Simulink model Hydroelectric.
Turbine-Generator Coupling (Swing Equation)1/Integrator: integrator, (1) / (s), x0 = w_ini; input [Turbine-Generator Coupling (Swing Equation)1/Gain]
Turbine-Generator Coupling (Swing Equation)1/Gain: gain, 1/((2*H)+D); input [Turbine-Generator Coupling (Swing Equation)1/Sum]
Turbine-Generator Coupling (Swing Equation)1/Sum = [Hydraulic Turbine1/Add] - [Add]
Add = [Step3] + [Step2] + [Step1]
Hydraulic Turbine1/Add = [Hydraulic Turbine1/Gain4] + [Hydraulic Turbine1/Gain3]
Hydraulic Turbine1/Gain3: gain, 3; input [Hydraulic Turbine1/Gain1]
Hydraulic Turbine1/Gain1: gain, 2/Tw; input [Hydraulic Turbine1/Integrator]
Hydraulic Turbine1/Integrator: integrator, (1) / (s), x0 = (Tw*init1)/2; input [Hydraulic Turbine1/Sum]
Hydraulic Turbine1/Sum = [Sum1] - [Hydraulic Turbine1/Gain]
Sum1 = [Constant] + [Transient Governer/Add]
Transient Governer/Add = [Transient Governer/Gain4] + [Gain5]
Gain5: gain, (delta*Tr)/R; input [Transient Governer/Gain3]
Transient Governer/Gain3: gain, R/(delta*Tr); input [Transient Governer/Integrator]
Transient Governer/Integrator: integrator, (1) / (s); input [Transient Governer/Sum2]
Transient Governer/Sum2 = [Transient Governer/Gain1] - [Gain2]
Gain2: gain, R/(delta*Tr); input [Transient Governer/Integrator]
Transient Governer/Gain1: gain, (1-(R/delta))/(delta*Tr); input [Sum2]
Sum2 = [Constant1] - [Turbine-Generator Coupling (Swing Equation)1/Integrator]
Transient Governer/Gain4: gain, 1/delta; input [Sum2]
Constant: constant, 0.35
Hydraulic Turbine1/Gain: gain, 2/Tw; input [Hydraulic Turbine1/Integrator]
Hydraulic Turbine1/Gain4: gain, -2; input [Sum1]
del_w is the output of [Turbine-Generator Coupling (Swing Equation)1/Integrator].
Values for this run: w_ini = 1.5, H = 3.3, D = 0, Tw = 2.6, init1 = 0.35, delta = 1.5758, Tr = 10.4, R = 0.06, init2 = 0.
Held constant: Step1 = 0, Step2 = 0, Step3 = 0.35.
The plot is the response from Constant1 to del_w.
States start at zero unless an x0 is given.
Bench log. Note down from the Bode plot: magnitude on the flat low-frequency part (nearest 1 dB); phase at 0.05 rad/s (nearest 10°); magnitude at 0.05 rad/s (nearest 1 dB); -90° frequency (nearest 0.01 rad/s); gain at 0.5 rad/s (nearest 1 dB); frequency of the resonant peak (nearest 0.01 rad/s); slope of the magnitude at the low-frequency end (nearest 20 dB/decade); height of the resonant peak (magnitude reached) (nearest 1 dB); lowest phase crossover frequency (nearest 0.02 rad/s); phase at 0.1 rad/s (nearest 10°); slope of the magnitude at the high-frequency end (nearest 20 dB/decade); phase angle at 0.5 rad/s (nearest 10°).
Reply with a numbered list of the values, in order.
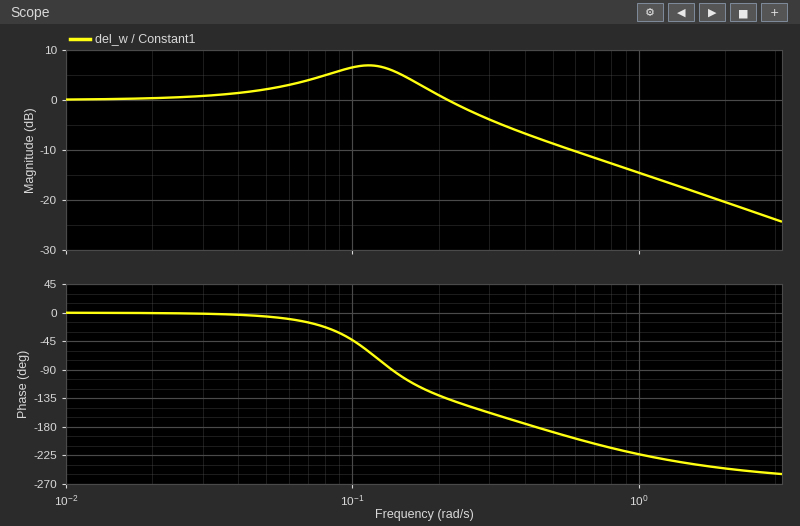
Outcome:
1. 0 dB
2. -10°
3. 2 dB
4. 0.14 rad/s
5. -9 dB
6. 0.11 rad/s
7. 0 dB/decade
8. 7 dB
9. 0.44 rad/s
10. -40°
11. -20 dB/decade
12. -190°
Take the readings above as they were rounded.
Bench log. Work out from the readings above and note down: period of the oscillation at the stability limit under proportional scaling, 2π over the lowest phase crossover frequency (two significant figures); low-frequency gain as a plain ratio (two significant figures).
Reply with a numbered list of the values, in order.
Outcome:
1. 14 s
2. 1.0
